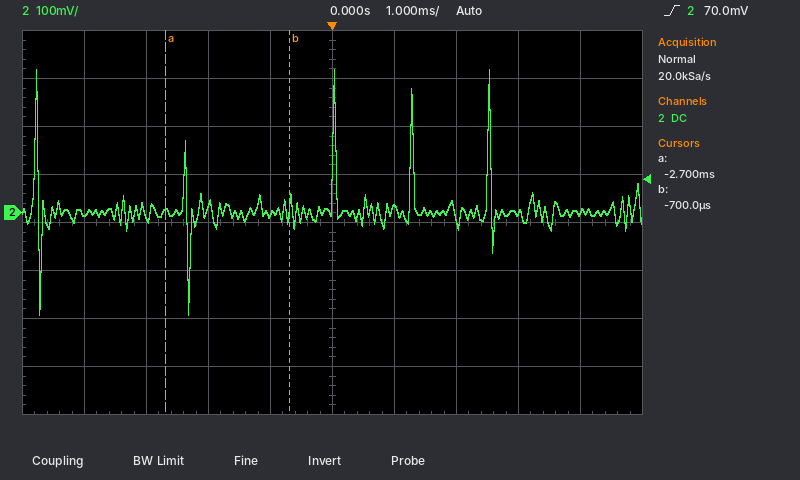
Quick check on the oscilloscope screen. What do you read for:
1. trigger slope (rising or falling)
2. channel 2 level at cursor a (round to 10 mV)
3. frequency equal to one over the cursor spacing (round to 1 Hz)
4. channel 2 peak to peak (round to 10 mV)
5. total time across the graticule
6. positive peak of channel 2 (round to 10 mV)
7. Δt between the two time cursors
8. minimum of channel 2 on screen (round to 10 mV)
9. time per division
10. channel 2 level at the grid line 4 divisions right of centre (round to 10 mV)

rising
0 mV
500 Hz
510 mV
10 ms
300 mV
2.0 ms
-210 mV
1 ms
0 mV
